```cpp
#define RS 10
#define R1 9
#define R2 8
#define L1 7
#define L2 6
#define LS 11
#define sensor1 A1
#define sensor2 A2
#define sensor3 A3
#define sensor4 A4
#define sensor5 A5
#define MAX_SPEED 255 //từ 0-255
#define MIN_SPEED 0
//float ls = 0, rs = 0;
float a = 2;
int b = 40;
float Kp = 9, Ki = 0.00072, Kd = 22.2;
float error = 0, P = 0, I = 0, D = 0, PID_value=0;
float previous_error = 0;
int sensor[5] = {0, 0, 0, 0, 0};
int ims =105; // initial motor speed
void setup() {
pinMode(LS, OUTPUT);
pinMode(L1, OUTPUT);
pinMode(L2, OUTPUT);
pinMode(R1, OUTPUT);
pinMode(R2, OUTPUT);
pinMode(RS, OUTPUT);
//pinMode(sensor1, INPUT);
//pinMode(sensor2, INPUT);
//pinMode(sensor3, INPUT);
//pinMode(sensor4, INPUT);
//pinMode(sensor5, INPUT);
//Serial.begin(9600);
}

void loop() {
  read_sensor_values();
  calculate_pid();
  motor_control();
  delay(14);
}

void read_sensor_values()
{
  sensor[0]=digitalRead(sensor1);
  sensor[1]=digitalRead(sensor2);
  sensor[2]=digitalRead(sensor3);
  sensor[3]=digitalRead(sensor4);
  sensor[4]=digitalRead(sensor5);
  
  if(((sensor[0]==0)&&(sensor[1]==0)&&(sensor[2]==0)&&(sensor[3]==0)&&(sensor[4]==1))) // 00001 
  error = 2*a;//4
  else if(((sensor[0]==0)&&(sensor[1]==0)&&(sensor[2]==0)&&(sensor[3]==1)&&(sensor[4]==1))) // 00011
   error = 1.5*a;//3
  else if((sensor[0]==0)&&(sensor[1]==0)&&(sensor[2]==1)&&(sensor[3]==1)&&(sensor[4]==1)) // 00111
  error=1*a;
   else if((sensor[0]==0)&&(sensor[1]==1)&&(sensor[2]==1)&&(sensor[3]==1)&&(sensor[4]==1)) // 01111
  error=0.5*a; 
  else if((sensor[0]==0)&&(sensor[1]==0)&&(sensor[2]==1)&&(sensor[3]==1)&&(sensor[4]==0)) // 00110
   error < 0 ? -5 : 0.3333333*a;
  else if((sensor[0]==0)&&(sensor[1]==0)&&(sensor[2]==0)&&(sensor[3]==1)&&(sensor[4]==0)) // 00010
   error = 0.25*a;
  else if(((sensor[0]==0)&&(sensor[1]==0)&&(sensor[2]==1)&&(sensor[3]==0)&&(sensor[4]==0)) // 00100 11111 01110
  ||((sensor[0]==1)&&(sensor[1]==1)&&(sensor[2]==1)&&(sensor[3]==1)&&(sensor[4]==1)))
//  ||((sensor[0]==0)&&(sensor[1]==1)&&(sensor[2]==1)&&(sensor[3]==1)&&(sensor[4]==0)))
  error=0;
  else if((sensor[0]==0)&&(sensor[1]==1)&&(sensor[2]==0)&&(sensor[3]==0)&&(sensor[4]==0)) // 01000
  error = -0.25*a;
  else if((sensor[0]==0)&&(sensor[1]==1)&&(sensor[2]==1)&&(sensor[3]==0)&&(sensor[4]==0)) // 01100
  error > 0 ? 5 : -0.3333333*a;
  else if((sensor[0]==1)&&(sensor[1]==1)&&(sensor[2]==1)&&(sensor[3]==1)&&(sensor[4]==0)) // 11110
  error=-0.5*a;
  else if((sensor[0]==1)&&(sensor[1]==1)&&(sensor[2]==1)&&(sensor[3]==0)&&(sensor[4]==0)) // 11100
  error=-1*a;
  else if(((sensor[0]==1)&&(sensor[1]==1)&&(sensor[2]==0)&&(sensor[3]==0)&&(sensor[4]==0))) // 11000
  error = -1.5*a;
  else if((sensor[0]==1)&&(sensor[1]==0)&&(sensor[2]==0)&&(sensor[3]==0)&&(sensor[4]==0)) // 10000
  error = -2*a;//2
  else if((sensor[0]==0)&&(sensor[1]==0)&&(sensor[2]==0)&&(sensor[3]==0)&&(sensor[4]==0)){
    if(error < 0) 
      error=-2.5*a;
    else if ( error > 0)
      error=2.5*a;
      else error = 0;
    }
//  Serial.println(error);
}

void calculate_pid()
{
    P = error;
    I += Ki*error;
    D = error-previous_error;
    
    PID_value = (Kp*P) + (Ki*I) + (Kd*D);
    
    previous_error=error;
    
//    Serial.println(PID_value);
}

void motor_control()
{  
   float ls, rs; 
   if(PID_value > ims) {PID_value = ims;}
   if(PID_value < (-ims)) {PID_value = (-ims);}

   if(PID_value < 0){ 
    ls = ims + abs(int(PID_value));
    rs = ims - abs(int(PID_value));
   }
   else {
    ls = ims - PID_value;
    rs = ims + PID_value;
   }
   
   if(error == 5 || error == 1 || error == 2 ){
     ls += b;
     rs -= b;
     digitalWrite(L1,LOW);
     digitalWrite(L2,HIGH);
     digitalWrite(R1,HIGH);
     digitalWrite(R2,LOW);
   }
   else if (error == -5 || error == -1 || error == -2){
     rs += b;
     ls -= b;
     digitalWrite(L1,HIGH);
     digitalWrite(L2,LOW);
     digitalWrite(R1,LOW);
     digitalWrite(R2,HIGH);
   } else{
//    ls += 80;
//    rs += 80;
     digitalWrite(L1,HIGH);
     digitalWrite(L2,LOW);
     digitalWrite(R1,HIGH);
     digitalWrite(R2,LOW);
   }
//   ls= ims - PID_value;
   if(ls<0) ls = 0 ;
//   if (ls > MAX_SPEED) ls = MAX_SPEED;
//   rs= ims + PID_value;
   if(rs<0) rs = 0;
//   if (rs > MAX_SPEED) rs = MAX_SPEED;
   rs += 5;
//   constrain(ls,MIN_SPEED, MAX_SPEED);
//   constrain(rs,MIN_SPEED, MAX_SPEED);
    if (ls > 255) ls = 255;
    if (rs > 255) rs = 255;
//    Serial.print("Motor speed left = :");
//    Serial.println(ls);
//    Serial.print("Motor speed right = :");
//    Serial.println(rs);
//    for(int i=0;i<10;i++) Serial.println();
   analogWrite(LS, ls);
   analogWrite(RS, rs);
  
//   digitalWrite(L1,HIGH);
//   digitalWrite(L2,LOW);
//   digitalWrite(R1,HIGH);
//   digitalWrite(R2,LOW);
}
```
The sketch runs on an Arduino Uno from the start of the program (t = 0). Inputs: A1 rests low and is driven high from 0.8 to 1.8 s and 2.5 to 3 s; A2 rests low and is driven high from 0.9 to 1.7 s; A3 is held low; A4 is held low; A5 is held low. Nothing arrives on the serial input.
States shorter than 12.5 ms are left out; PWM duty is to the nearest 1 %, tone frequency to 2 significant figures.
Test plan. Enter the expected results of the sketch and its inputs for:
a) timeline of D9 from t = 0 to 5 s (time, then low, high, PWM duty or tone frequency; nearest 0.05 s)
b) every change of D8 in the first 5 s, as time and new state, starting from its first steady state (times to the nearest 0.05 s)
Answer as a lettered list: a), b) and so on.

a) 0 s high; 1.8 s low; 2.5 s high; 3 s low
b) 0 s low; 1.8 s high; 2.5 s low; 3 s high
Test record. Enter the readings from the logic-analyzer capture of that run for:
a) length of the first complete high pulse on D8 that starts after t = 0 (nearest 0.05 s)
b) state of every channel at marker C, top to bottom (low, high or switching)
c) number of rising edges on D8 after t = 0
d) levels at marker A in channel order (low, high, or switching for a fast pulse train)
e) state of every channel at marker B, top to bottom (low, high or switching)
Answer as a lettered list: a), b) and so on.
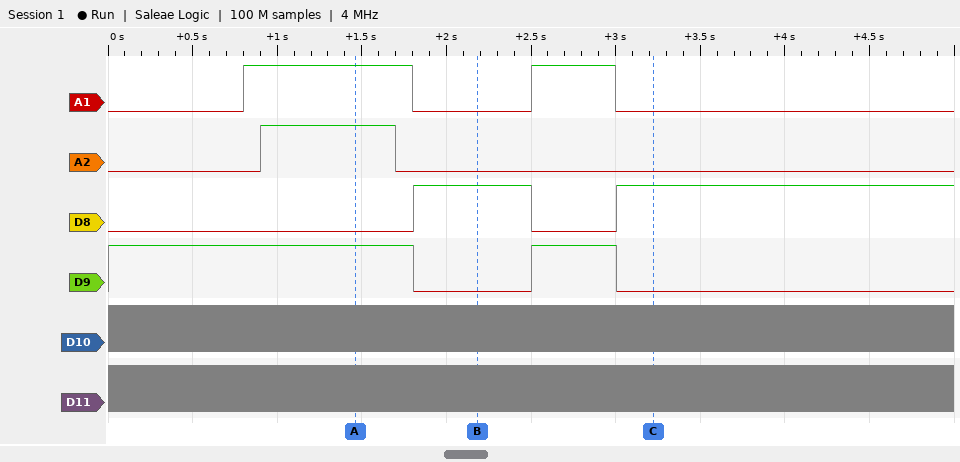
a) 0.70 s
b) A1 low, A2 low, D8 high, D9 low, D10 switching, D11 switching
c) 2
d) A1 high, A2 high, D8 low, D9 high, D10 switching, D11 switching
e) A1 low, A2 low, D8 high, D9 low, D10 switching, D11 switching
